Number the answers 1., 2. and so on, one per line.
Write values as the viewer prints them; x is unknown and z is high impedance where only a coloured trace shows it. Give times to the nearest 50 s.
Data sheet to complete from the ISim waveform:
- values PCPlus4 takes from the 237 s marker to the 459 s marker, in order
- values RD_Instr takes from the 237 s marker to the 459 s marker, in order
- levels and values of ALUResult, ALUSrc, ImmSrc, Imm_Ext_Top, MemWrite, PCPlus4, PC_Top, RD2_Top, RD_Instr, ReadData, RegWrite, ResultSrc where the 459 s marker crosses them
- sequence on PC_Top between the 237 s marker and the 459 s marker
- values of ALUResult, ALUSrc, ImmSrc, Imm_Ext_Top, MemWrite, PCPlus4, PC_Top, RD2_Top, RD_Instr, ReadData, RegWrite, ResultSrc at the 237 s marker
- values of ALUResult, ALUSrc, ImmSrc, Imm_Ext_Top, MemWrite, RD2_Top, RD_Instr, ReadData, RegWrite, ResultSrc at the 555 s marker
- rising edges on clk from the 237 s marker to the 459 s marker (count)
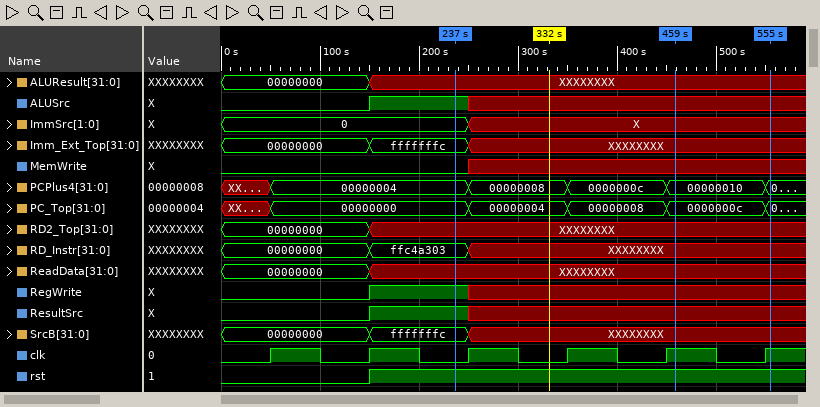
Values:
1. 00000004, 00000008, 0000000c, 00000010
2. ffc4a303, XXXXXXXX
3. ALUResult=XXXXXXXX, ALUSrc=x, ImmSrc=X, Imm_Ext_Top=XXXXXXXX, MemWrite=x, PCPlus4=00000010, PC_Top=0000000c, RD2_Top=XXXXXXXX, RD_Instr=XXXXXXXX, ReadData=XXXXXXXX, RegWrite=x, ResultSrc=x
4. 00000000, 00000004, 00000008, 0000000c
5. ALUResult=XXXXXXXX, ALUSrc=1, ImmSrc=0, Imm_Ext_Top=fffffffc, MemWrite=0, PCPlus4=00000004, PC_Top=00000000, RD2_Top=XXXXXXXX, RD_Instr=ffc4a303, ReadData=XXXXXXXX, RegWrite=1, ResultSrc=1
6. ALUResult=XXXXXXXX, ALUSrc=x, ImmSrc=X, Imm_Ext_Top=XXXXXXXX, MemWrite=x, RD2_Top=XXXXXXXX, RD_Instr=XXXXXXXX, ReadData=XXXXXXXX, RegWrite=x, ResultSrc=x
7. 3
